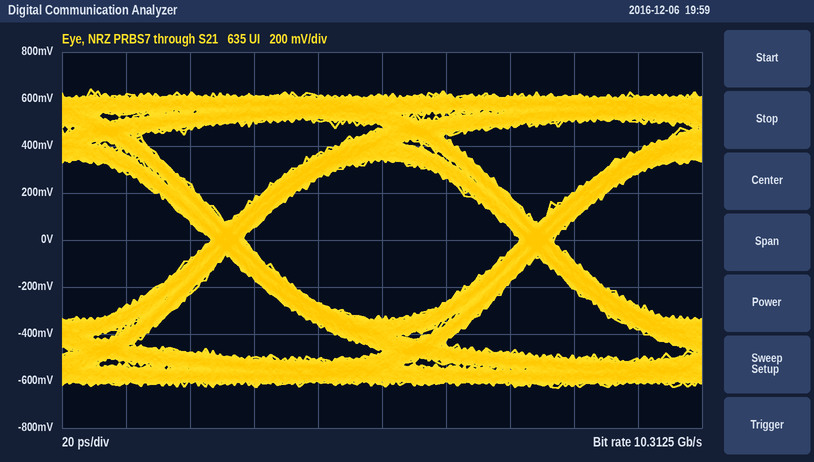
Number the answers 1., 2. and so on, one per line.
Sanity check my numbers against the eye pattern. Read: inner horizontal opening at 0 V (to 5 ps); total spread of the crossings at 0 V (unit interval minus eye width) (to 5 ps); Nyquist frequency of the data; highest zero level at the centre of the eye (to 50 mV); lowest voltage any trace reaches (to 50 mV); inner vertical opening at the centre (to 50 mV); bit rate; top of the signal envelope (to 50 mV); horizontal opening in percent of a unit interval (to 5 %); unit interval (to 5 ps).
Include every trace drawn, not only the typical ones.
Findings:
1. 85 ps
2. 10 ps
3. 5.15625 GHz
4. -350 mV
5. -650 mV
6. 700 mV
7. 10.3125 Gb/s
8. 650 mV
9. 90 %
10. 95 ps
